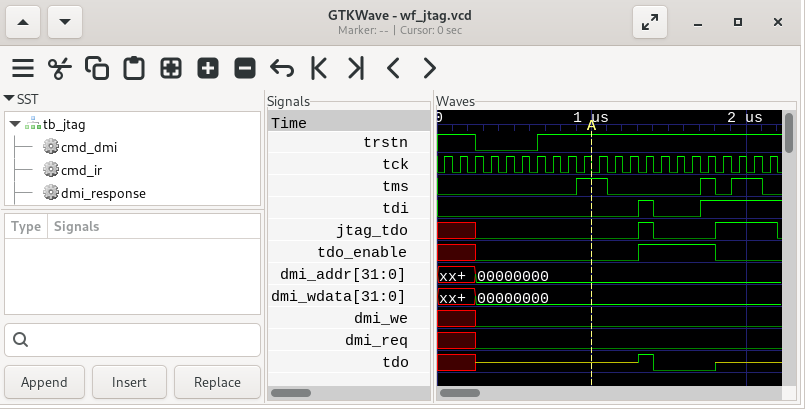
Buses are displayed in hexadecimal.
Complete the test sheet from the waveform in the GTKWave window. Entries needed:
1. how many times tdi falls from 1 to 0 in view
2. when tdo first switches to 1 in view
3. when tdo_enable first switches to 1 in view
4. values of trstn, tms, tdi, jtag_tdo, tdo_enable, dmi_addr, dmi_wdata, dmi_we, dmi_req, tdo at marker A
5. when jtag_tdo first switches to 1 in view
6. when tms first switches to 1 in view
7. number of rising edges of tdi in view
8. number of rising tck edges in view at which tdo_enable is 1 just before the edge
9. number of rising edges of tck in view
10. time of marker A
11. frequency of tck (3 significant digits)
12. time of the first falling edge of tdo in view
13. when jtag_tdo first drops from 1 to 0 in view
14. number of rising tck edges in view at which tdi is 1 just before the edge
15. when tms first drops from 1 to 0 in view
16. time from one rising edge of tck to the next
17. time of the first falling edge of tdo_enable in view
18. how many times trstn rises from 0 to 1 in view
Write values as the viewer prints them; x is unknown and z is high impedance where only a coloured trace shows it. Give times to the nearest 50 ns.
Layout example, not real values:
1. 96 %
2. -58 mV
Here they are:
1. 1
2. 1300 ns
3. 1300 ns
4. trstn=1, tms=1, tdi=0, jtag_tdo=0, tdo_enable=0, dmi_addr=00000000, dmi_wdata=00000000, dmi_we=0, dmi_req=0, tdo=z
5. 1300 ns
6. 900 ns
7. 2
8. 5
9. 22
10. 1000 ns
11. 10.0 MHz
12. 1400 ns
13. 1400 ns
14. 6
15. 1100 ns
16. 100 ns
17. 1800 ns
18. 1
